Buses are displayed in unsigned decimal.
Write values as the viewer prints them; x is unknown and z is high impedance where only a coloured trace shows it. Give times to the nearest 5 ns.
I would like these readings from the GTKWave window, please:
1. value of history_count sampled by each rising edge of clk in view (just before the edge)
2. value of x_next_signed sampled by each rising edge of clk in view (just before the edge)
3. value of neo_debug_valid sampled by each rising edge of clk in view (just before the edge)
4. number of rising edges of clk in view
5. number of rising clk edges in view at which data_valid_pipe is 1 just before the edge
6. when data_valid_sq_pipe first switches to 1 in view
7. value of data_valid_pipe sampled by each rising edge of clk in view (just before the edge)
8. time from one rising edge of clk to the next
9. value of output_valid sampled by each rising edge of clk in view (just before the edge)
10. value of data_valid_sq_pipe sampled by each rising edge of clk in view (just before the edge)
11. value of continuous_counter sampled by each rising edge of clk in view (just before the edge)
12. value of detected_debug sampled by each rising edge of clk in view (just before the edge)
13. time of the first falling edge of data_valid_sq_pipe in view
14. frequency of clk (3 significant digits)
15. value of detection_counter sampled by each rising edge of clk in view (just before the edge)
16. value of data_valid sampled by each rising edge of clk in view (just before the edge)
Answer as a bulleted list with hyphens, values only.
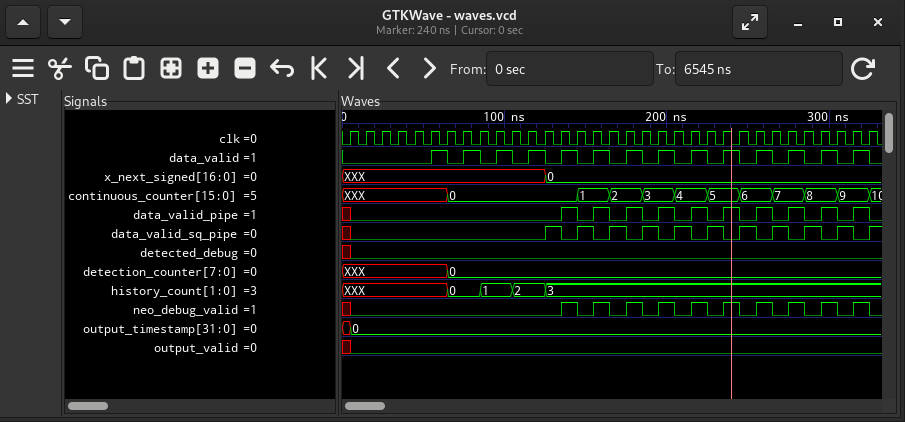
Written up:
- XXX, XXX, XXX, XXX, XXX, XXX, XXX, 0, 0, 1, 1, 2, 2, 3, 3, 3, 3, 3, 3, 3, 3, 3, 3, 3, 3, 3, 3, 3, 3, 3, 3, 3, 3
- XXX, XXX, XXX, XXX, XXX, XXX, XXX, XXX, XXX, XXX, XXX, XXX, XXX, 0, 0, 0, 0, 0, 0, 0, 0, 0, 0, 0, 0, 0, 0, 0, 0, 0, 0, 0, 0
- x 0 0 0 0 0 0 0 0 0 0 0 0 0 1 0 1 0 1 0 1 0 1 0 1 0 1 0 1 0 1 0 1
- 33
- 10
- 125 ns
- x 0 0 0 0 0 0 0 0 0 0 0 0 0 1 0 1 0 1 0 1 0 1 0 1 0 1 0 1 0 1 0 1
- 10 ns
- x 0 0 0 0 0 0 0 0 0 0 0 0 0 0 0 0 0 0 0 0 0 0 0 0 0 0 0 0 0 0 0 0
- x 0 0 0 0 0 0 0 0 0 0 0 0 1 0 1 0 1 0 1 0 1 0 1 0 1 0 1 0 1 0 1 0
- XXX, XXX, XXX, XXX, XXX, XXX, XXX, 0, 0, 0, 0, 0, 0, 0, 0, 1, 1, 2, 2, 3, 3, 4, 4, 5, 5, 6, 6, 7, 7, 8, 8, 9, 9
- x 0 0 0 0 0 0 0 0 0 0 0 0 0 0 0 0 0 0 0 0 0 0 0 0 0 0 0 0 0 0 0 0
- 135 ns
- 100 MHz
- XXX, XXX, XXX, XXX, XXX, XXX, XXX, 0, 0, 0, 0, 0, 0, 0, 0, 0, 0, 0, 0, 0, 0, 0, 0, 0, 0, 0, 0, 0, 0, 0, 0, 0, 0
- 0 0 0 0 0 0 1 0 1 0 1 0 1 0 1 0 1 0 1 0 1 0 1 0 1 0 1 0 1 0 1 0 1
